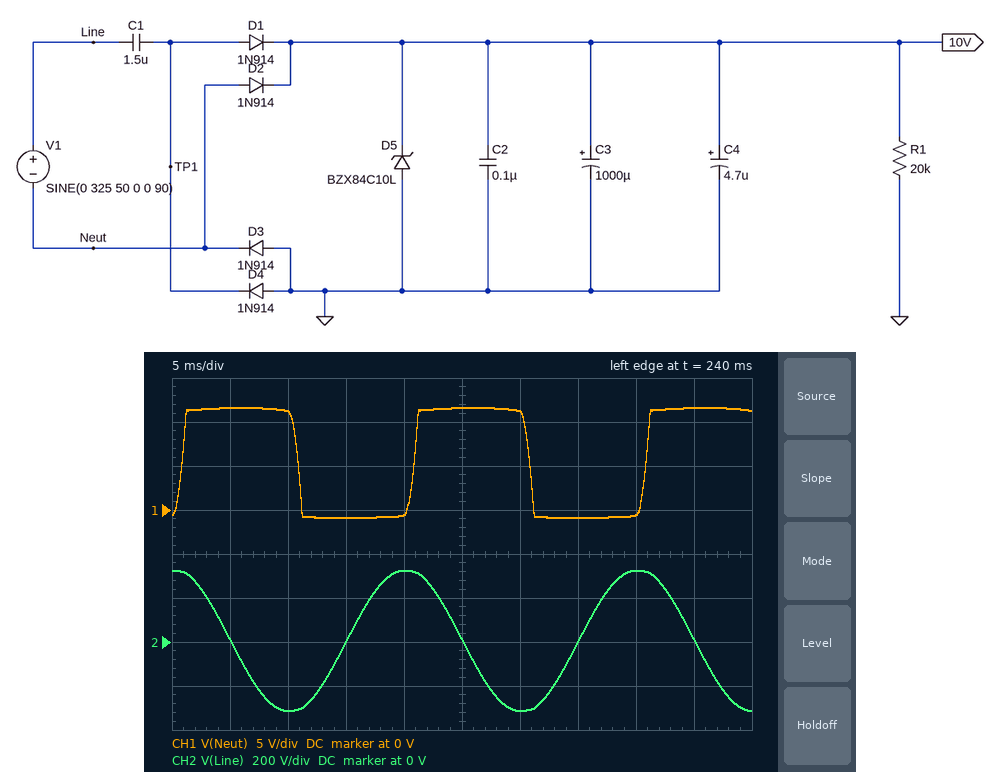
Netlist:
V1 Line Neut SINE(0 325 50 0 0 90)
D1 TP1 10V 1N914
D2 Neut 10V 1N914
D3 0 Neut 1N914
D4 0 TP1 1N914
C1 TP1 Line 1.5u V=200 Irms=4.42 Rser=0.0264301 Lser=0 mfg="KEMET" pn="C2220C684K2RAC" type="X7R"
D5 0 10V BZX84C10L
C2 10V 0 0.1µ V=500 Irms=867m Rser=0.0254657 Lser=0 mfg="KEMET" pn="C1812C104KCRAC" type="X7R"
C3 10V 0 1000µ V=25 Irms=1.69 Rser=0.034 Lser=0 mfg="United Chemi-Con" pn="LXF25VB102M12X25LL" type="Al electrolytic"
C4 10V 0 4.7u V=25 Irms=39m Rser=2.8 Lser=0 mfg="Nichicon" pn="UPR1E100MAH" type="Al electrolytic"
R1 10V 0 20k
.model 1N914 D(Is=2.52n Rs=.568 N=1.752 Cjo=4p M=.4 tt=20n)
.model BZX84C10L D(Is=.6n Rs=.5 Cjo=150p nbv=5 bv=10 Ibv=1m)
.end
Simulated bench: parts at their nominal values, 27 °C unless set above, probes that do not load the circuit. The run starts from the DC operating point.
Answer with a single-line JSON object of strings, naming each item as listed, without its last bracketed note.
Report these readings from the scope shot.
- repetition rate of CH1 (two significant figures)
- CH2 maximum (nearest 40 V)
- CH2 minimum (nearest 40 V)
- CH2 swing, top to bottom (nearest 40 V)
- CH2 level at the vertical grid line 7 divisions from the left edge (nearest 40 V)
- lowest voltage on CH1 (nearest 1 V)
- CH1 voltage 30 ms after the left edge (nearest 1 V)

{"repetition rate of CH1": "50 Hz", "CH2 maximum": "320 V", "CH2 minimum": "-320 V", "CH2 swing, top to bottom": "640 V", "CH2 level at the vertical grid line 7 divisions from the left edge": "0 V", "lowest voltage on CH1": "-1 V", "CH1 voltage 30 ms after the left edge": "11 V"}
